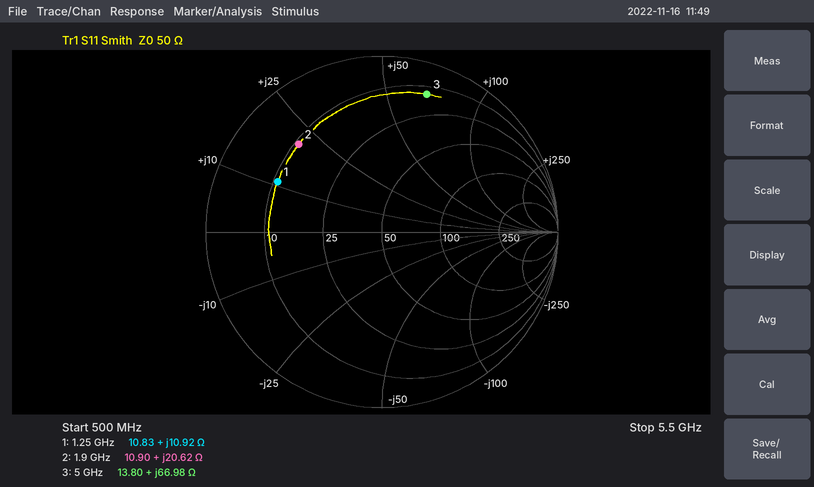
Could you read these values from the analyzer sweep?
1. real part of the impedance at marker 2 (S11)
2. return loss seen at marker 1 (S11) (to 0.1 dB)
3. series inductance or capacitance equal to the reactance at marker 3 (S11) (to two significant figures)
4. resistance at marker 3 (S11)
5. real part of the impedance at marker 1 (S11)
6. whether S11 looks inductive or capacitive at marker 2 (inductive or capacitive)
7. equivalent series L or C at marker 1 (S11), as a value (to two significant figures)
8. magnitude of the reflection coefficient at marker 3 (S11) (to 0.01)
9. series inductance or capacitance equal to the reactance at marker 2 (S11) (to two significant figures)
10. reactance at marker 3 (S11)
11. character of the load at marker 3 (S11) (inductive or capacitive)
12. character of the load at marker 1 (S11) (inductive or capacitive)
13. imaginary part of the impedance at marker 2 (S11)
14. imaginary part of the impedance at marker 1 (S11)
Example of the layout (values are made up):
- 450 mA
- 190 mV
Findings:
- 10.90 Ω
- 3.6 dB
- 2.1 nH
- 13.80 Ω
- 10.83 Ω
- inductive
- 1.4 nH
- 0.82
- 1.7 nH
- +66.98 Ω
- inductive
- inductive
- +20.62 Ω
- +10.92 Ω
